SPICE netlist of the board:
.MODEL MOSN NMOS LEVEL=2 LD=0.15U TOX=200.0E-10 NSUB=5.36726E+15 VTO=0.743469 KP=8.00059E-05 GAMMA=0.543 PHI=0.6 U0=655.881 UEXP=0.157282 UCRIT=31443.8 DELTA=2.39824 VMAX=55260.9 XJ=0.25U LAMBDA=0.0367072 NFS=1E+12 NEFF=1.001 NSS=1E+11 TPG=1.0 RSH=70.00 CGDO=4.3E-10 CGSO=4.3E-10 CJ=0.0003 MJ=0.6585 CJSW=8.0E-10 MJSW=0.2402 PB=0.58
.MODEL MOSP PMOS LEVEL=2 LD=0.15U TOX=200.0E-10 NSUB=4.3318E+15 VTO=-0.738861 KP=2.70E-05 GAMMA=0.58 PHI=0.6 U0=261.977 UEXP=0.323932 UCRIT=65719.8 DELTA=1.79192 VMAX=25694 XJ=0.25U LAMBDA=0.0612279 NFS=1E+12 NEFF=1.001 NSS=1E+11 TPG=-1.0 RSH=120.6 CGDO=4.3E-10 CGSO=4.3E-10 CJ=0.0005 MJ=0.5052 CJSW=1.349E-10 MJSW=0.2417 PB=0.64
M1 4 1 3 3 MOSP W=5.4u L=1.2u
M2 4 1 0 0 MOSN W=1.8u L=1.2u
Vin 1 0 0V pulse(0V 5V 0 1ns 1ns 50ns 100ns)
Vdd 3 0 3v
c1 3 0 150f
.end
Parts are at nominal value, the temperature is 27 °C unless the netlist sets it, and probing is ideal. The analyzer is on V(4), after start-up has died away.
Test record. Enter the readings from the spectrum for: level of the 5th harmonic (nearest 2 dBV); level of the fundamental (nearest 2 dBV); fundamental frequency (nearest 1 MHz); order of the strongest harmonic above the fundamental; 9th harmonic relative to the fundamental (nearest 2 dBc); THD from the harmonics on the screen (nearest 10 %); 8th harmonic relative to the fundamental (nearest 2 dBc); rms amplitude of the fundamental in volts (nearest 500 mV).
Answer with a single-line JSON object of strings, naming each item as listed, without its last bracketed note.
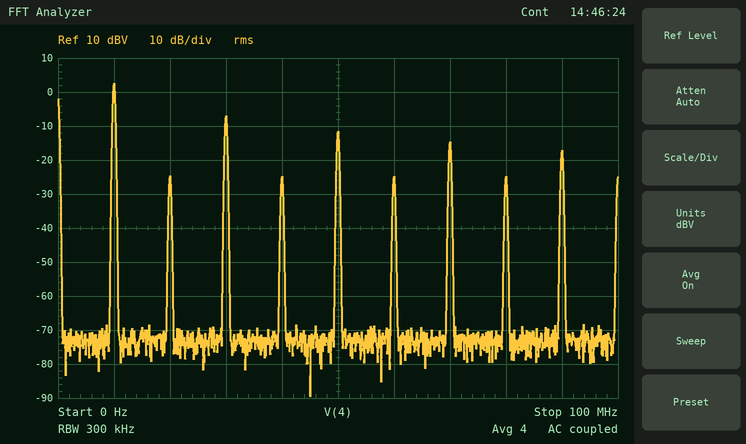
{"level of the 5th harmonic": "-12 dBV", "level of the fundamental": "2 dBV", "fundamental frequency": "10 MHz", "order of the strongest harmonic above the fundamental": "3", "9th harmonic relative to the fundamental": "-20 dBc", "THD from the harmonics on the screen": "40 %", "8th harmonic relative to the fundamental": "-28 dBc", "rms amplitude of the fundamental in volts": "1.5 V"}
